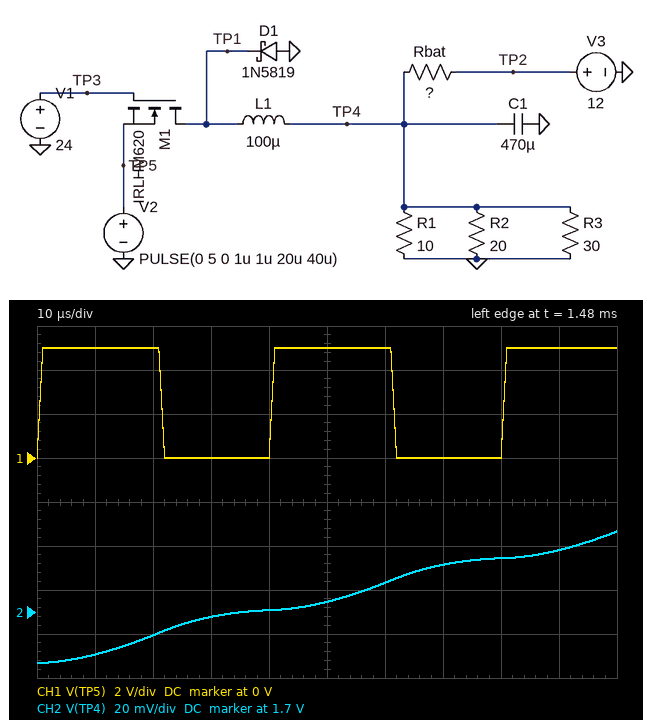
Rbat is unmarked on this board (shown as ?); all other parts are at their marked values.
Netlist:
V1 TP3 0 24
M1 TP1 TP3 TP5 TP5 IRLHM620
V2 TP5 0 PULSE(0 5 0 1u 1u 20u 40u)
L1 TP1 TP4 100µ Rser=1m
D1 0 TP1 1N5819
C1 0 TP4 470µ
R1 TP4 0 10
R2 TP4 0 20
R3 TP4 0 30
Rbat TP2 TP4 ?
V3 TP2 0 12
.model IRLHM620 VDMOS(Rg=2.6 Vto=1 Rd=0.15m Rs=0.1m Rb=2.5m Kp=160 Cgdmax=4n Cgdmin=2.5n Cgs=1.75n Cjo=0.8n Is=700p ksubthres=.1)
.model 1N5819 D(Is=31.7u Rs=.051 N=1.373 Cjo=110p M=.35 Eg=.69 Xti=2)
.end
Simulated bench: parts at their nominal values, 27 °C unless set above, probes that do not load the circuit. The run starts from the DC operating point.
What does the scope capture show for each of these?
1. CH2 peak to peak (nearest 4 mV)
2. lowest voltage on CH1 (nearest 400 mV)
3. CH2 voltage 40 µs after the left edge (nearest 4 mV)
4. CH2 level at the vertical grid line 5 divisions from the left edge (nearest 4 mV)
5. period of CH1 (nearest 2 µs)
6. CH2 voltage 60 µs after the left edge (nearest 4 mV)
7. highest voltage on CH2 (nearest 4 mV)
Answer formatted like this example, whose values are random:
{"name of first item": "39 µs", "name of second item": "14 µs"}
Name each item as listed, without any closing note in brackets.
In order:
{"CH2 peak to peak": "60 mV", "lowest voltage on CH1": "0 V", "CH2 voltage 40 µs after the left edge": "1.700 V", "CH2 level at the vertical grid line 5 divisions from the left edge": "1.704 V", "period of CH1": "40 µs", "CH2 voltage 60 µs after the left edge": "1.712 V", "highest voltage on CH2": "1.736 V"}
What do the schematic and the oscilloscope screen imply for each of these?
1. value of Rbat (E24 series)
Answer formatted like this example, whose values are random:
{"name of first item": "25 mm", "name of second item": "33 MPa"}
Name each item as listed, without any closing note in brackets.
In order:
{"value of Rbat": "0.047 Ω"}
